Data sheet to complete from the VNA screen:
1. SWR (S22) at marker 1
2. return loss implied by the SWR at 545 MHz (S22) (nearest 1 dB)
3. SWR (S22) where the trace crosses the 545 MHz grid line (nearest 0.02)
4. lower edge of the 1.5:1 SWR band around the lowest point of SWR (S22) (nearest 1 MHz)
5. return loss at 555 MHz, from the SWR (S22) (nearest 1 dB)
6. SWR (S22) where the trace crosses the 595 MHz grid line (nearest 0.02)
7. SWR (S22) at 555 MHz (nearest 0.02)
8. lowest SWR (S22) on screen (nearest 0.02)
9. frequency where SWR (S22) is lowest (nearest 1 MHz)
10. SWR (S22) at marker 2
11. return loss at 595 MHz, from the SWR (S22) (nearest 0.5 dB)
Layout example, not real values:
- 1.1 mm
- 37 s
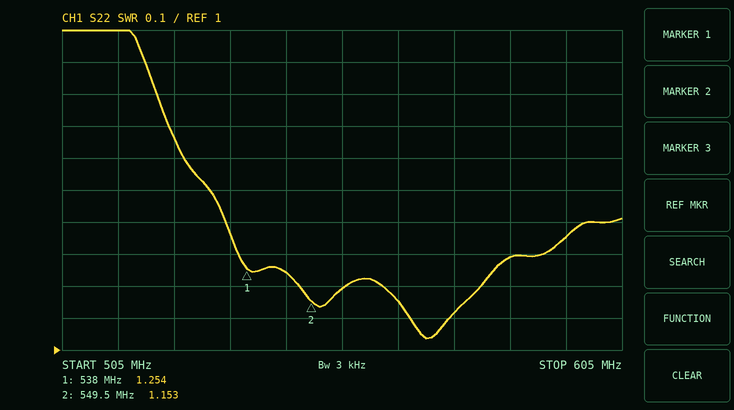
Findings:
- 1.254
- 19 dB
- 1.24
- 531 MHz
- 21 dB
- 1.36
- 1.20
- 1.04
- 570 MHz
- 1.153
- 16.5 dB
